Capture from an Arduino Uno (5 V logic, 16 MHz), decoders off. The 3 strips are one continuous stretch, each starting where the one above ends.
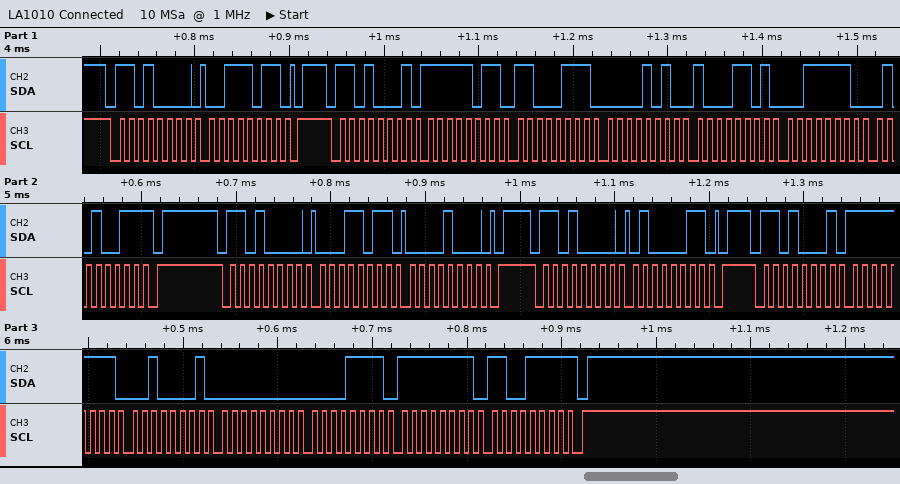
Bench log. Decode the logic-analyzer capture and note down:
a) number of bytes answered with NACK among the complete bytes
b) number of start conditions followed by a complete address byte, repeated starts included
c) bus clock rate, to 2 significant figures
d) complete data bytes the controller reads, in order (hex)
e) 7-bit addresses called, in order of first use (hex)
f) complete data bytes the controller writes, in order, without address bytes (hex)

2
5
100 kHz
FB C7 0A 8D 3E 53 FF 21 00 0F FF CF
0x68
3B 1B 08 43
